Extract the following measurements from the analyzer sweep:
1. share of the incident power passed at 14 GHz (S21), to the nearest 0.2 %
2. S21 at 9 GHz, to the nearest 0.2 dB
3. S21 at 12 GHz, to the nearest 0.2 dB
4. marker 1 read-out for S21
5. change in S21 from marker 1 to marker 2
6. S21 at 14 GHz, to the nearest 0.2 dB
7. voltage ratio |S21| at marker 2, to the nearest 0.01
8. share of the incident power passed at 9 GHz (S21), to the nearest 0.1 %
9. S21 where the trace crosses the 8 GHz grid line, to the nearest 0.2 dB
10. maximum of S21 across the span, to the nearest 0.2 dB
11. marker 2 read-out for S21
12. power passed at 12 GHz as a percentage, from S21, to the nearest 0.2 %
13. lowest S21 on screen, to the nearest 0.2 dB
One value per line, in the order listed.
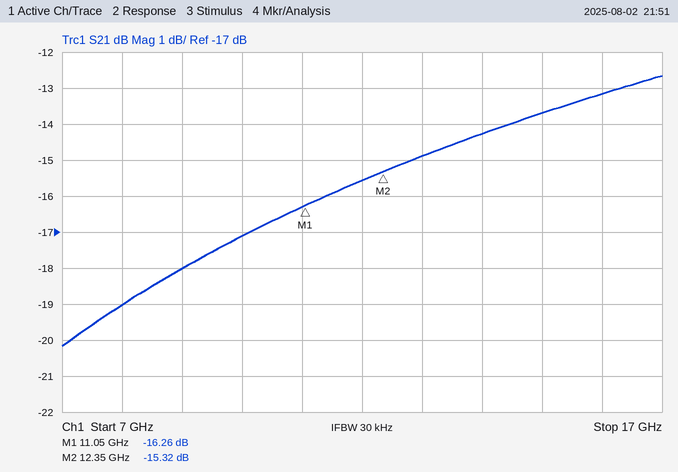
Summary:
3.8 %
-18.0 dB
-15.6 dB
-16.26 dB
0.94 dB
-14.2 dB
0.17
1.6 %
-19.0 dB
-12.6 dB
-15.32 dB
2.8 %
-20.2 dB
